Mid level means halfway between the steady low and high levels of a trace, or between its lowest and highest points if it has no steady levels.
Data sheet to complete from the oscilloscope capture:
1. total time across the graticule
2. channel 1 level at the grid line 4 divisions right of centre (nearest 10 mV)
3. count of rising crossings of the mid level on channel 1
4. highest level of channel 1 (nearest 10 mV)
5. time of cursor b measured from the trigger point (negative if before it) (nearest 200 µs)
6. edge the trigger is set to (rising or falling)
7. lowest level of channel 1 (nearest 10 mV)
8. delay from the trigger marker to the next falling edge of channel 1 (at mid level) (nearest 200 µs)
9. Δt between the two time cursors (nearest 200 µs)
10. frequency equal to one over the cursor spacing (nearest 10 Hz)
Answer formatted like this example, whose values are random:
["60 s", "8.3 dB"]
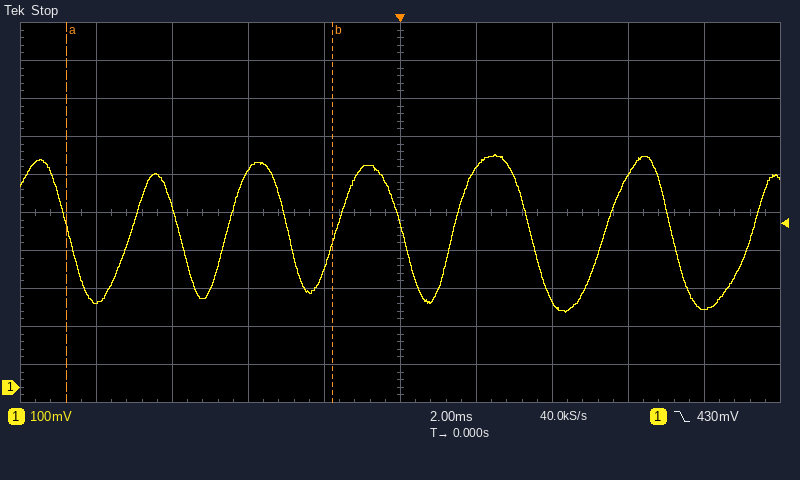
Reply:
["20 ms", "210 mV", "6", "610 mV", "-1.8 ms", "falling", "200 mV", "3.4 ms", "7.0 ms", "140 Hz"]
